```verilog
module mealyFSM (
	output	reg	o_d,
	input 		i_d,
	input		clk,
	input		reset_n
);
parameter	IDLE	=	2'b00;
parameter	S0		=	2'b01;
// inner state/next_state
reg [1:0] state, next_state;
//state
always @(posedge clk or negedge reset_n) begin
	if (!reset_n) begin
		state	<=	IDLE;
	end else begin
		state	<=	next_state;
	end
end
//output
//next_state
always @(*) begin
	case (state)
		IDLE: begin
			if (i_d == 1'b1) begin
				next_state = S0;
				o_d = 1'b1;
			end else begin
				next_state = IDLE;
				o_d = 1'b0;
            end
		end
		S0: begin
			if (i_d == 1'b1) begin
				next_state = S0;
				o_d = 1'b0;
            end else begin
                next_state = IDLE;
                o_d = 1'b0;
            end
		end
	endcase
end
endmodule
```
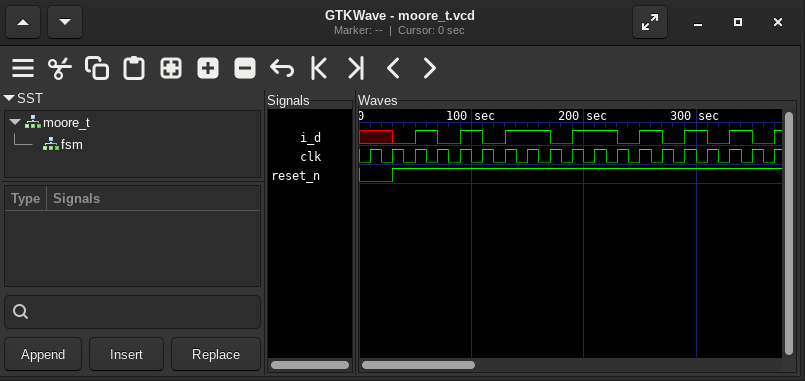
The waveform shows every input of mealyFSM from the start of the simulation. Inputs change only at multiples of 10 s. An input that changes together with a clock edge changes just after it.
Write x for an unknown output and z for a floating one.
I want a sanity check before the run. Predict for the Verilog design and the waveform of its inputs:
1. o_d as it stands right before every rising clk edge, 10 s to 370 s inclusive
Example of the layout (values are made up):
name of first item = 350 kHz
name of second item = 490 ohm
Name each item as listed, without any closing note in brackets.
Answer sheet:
o_d as it stands right before every rising clk edge, 10 s to 370 s inclusive = 0 0 0 1 0 1 0 1 0 0 1 0 0 1 0 1 0 1 0
